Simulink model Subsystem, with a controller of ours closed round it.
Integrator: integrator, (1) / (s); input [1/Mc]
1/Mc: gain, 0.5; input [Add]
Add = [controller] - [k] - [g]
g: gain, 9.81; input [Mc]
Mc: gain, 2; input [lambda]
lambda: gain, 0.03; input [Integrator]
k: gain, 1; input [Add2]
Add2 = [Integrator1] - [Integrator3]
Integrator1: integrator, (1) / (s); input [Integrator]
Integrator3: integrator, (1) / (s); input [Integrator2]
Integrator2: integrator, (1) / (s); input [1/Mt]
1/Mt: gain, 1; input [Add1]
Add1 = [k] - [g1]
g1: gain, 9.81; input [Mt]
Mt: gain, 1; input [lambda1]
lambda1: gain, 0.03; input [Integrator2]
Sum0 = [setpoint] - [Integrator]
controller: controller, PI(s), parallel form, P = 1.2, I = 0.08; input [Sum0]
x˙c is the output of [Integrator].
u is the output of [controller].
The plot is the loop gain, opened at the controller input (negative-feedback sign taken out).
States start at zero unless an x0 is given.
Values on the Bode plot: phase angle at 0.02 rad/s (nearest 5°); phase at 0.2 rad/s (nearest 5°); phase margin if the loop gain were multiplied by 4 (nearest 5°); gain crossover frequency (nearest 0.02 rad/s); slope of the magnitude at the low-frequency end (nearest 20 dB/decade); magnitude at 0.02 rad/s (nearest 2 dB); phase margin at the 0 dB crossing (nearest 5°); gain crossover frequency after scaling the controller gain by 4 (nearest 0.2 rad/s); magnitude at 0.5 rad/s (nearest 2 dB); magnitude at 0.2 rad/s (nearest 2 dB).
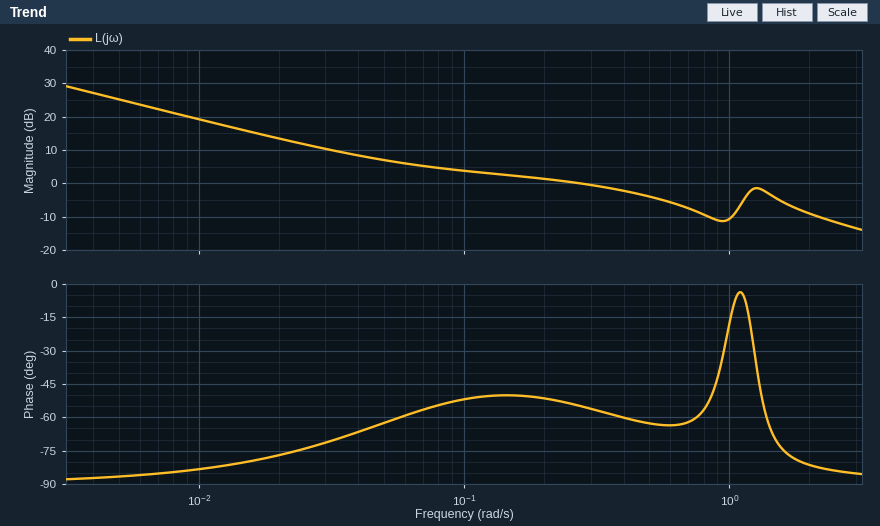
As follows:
-75°
-50°
95°
0.28 rad/s
-20 dB/decade
14 dB
125°
2.6 rad/s
-4 dB
2 dB
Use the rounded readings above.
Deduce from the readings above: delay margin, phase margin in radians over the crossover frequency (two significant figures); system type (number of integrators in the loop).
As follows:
7.8 s
1
